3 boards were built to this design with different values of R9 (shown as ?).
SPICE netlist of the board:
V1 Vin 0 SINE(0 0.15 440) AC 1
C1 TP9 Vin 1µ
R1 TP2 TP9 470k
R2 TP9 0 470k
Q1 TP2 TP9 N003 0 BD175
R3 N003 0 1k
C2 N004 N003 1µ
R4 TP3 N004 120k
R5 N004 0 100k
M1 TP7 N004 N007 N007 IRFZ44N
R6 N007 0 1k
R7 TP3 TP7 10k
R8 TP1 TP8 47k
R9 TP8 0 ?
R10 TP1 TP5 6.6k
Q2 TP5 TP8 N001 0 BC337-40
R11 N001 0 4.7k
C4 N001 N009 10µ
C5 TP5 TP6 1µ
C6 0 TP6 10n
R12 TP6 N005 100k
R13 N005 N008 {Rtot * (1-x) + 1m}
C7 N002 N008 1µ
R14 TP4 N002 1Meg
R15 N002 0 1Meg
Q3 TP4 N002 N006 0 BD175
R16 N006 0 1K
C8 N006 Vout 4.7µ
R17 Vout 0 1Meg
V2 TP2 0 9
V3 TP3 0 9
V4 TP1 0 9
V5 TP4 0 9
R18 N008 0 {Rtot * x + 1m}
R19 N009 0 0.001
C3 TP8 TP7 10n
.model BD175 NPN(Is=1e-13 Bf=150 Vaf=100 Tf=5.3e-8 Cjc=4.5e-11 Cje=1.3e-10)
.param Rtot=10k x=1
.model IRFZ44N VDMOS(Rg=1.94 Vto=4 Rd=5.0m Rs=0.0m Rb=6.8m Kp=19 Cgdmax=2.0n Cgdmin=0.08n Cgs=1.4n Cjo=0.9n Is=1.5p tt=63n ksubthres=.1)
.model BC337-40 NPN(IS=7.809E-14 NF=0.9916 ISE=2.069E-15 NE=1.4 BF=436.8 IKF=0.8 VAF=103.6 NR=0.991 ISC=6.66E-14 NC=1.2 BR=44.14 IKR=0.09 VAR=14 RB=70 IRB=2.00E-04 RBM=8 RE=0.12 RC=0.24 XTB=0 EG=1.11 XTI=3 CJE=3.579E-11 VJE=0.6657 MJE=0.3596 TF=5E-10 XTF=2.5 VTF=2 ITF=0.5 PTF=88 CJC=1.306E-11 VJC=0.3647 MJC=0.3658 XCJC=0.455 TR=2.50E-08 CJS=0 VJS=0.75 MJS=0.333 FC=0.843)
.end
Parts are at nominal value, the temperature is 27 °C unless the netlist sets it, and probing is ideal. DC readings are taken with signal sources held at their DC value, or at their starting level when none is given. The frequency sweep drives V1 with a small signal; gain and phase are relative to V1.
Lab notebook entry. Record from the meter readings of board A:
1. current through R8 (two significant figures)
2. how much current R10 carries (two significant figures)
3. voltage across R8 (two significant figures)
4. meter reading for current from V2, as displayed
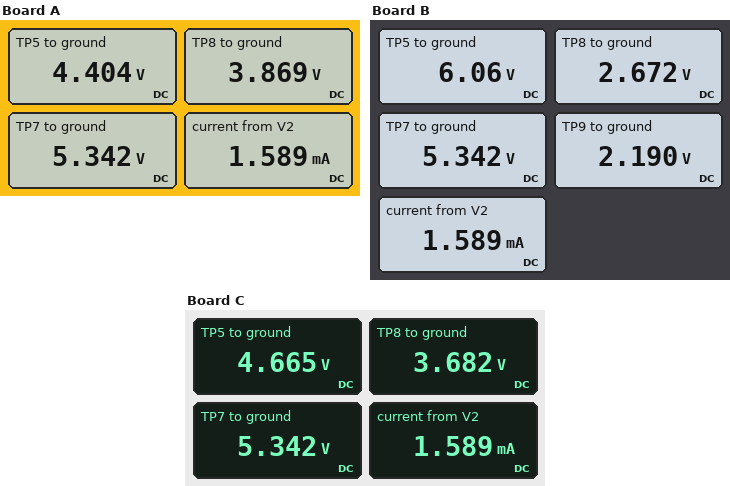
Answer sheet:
110 µA
700 µA
5.1 V
1.589 mA
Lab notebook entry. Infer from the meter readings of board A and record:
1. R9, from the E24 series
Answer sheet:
36 kΩ
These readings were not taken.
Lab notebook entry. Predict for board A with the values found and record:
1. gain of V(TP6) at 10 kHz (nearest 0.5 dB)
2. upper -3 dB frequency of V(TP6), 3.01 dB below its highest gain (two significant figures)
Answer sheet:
43.0 dB
4.0 kHz
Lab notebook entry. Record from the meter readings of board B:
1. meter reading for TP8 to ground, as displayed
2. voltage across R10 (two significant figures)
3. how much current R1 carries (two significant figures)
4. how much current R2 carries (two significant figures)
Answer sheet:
2.672 V
2.9 V
14 µA
4.7 µA
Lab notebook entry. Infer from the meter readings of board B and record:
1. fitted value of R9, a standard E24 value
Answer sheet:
20 kΩ
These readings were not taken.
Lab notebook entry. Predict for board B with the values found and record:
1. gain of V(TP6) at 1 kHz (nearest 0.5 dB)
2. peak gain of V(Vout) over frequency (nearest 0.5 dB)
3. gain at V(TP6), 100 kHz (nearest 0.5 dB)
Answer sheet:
49.0 dB
28.0 dB
14.5 dB
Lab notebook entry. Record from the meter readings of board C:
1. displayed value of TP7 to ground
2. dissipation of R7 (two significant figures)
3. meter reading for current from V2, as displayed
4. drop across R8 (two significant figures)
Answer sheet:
5.342 V
1.3 mW
1.589 mA
5.3 V
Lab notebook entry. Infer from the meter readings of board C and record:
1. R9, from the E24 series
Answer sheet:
33 kΩ
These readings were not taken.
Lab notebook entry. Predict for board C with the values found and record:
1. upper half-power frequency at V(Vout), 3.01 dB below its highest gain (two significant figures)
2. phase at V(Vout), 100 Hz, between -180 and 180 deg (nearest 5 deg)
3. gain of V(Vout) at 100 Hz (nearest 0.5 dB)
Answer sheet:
4.0 kHz
140 deg
9.0 dB
